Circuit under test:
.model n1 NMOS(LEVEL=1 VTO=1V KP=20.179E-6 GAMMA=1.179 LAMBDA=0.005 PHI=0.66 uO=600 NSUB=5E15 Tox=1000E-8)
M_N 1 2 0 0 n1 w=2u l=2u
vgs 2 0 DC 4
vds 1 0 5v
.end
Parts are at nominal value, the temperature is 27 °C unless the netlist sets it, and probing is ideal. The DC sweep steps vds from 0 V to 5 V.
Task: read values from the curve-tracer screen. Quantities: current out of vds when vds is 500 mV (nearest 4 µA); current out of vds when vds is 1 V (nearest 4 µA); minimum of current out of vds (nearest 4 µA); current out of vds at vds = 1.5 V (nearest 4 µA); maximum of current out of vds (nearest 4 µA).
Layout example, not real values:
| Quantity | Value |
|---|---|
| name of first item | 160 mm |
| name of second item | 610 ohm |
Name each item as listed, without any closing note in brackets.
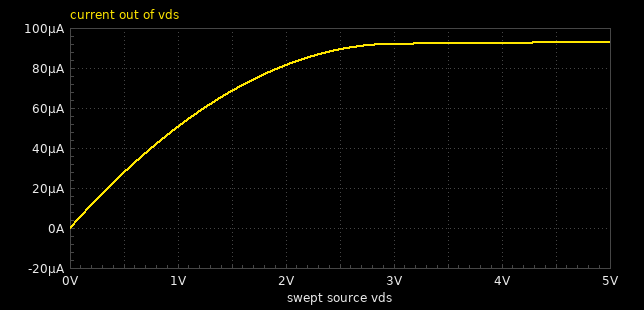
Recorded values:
| Quantity | Value |
|---|---|
| current out of vds when vds is 500 mV | 28 µA |
| current out of vds when vds is 1 V | 52 µA |
| minimum of current out of vds | 0 A |
| current out of vds at vds = 1.5 V | 68 µA |
| maximum of current out of vds | 92 µA |
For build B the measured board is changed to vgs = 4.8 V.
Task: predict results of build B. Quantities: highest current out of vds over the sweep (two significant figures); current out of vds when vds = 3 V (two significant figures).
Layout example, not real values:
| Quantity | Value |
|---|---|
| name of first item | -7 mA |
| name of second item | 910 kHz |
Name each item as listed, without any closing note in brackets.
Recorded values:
| Quantity | Value |
|---|---|
| highest current out of vds over the sweep | 150 µA |
| current out of vds when vds = 3 V | 140 µA |
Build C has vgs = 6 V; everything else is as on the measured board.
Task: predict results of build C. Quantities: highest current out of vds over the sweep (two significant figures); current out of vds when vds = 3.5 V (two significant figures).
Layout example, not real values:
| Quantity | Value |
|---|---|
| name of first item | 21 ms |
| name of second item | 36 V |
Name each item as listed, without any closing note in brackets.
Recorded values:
| Quantity | Value |
|---|---|
| highest current out of vds over the sweep | 260 µA |
| current out of vds when vds = 3.5 V | 230 µA |
